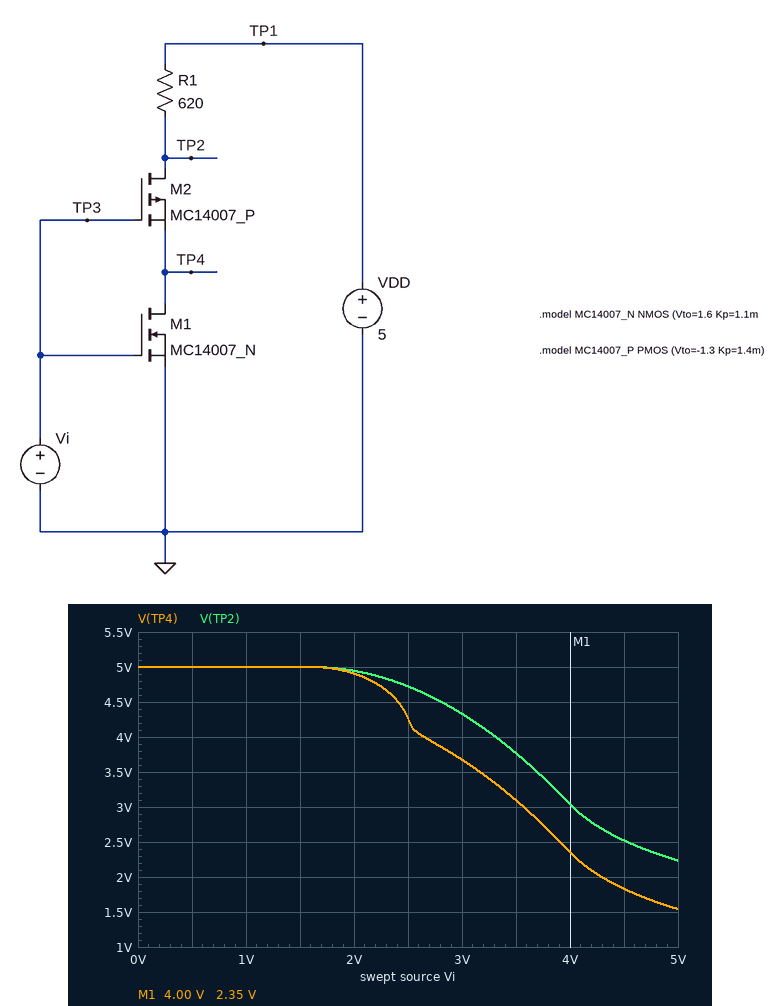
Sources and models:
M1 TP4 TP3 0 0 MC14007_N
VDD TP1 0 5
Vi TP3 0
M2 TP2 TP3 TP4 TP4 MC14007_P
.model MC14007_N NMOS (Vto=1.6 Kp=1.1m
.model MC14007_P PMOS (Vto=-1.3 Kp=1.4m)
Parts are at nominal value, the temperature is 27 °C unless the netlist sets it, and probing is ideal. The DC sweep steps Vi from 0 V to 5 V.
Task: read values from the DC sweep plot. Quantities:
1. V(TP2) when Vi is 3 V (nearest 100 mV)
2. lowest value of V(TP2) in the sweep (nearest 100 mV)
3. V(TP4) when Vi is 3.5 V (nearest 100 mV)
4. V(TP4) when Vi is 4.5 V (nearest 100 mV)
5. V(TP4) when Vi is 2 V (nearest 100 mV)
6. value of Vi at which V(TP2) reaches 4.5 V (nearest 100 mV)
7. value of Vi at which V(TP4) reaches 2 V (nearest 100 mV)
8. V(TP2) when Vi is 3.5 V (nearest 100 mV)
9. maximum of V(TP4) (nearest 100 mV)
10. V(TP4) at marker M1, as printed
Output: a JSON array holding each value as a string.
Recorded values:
["4.3 V", "2.2 V", "3.1 V", "1.8 V", "4.9 V", "2.8 V", "4.3 V", "3.8 V", "5.0 V", "2.35 V"]
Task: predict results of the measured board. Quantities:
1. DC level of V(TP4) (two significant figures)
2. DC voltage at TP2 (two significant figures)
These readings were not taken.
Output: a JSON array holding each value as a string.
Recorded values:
["5.0 V", "5.0 V"]
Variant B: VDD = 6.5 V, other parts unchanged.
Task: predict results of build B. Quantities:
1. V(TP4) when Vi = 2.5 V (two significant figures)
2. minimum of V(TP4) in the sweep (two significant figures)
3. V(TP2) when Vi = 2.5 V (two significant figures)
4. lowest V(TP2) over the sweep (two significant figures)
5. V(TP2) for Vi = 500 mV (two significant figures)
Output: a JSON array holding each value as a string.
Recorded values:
["6.1 V", "2.3 V", "6.2 V", "3.0 V", "6.5 V"]
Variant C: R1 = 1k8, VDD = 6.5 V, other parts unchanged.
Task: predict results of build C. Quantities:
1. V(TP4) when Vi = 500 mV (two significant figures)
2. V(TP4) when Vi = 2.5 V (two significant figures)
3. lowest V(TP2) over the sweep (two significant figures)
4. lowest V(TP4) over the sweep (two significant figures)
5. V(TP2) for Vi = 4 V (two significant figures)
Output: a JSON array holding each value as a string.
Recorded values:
["6.5 V", "5.5 V", "1.5 V", "840 mV", "2.0 V"]
